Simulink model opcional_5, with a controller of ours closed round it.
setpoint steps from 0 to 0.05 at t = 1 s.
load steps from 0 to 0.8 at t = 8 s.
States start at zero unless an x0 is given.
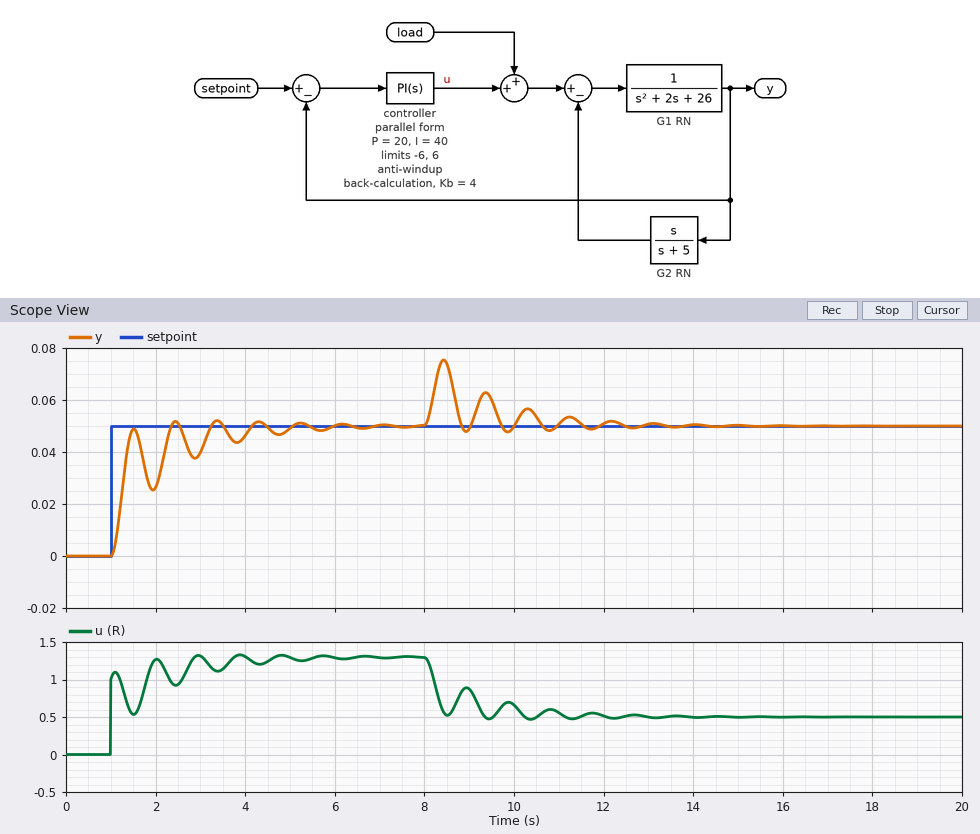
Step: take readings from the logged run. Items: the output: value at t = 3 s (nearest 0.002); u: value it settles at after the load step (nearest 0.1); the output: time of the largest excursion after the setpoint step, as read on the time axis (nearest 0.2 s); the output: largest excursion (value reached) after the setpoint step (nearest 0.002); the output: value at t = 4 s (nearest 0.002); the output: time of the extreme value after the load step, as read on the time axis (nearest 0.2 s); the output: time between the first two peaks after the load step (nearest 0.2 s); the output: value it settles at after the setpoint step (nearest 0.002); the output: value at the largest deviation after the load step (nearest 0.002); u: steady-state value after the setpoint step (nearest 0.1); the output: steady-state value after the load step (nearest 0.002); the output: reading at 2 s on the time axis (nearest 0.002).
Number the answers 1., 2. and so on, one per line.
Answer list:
1. 0.040
2. 0.5
3. 3.4 s
4. 0.052
5. 0.046
6. 8.4 s
7. 1.0 s
8. 0.050
9. 0.076
10. 1.3
11. 0.050
12. 0.026
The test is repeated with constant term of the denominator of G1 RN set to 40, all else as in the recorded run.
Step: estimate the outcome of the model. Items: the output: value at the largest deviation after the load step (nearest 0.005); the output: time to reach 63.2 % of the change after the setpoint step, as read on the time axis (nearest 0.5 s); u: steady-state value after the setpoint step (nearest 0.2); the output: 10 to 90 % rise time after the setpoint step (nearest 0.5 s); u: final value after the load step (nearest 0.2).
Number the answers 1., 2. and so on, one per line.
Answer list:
1. 0.070
2. 1.5 s
3. 2.0
4. 2.0 s
5. 1.2
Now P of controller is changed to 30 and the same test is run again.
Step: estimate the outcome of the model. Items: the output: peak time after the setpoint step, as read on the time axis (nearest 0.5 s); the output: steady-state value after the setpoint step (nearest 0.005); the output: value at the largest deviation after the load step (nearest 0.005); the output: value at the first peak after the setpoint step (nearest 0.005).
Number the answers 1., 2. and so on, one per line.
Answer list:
1. 1.5 s
2. 0.050
3. 0.070
4. 0.055
